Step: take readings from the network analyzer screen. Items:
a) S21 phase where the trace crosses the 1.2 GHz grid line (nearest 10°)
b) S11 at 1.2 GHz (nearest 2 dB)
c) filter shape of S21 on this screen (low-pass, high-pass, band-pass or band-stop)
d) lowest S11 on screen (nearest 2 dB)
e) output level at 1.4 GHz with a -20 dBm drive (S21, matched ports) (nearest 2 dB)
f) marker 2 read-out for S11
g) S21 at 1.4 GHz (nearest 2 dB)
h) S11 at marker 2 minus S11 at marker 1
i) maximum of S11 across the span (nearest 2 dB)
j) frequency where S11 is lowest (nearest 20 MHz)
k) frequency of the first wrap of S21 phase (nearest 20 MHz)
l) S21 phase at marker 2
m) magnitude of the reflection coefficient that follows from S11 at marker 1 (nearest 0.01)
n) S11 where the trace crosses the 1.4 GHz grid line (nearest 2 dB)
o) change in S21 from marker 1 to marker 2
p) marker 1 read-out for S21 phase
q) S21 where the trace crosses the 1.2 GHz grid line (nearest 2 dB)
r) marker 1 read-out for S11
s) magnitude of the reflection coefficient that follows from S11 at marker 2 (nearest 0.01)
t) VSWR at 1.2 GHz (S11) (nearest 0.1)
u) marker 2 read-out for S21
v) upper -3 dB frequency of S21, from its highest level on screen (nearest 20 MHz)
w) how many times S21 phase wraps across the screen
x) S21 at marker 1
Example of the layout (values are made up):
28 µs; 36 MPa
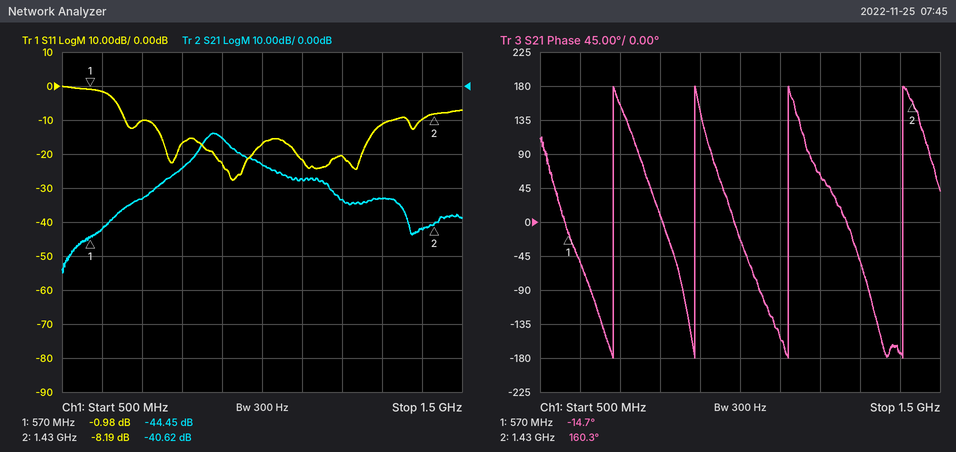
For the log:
60°; -20 dB; band-pass; -28 dB; -62 dBm; -8.19 dB; -42 dB; -7.21 dB; 0 dB; 920 MHz; 680 MHz; 160.3°; 0.89; -10 dB; 3.83 dB; -14.7°; -34 dB; -0.98 dB; 0.39; 1.2; -40.62 dB; 920 MHz; 4; -44.45 dB
